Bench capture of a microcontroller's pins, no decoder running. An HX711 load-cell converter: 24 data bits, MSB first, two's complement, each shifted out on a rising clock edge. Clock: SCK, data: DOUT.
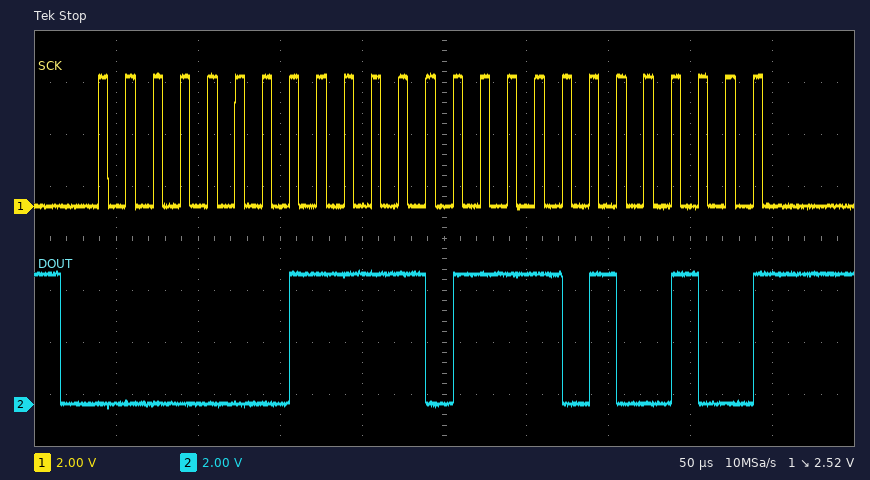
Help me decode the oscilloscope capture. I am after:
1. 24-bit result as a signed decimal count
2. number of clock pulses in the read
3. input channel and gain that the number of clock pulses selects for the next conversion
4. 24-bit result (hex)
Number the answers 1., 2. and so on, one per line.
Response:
1. 128932
2. 25
3. channel A, gain 128
4. 0x01F7A4
